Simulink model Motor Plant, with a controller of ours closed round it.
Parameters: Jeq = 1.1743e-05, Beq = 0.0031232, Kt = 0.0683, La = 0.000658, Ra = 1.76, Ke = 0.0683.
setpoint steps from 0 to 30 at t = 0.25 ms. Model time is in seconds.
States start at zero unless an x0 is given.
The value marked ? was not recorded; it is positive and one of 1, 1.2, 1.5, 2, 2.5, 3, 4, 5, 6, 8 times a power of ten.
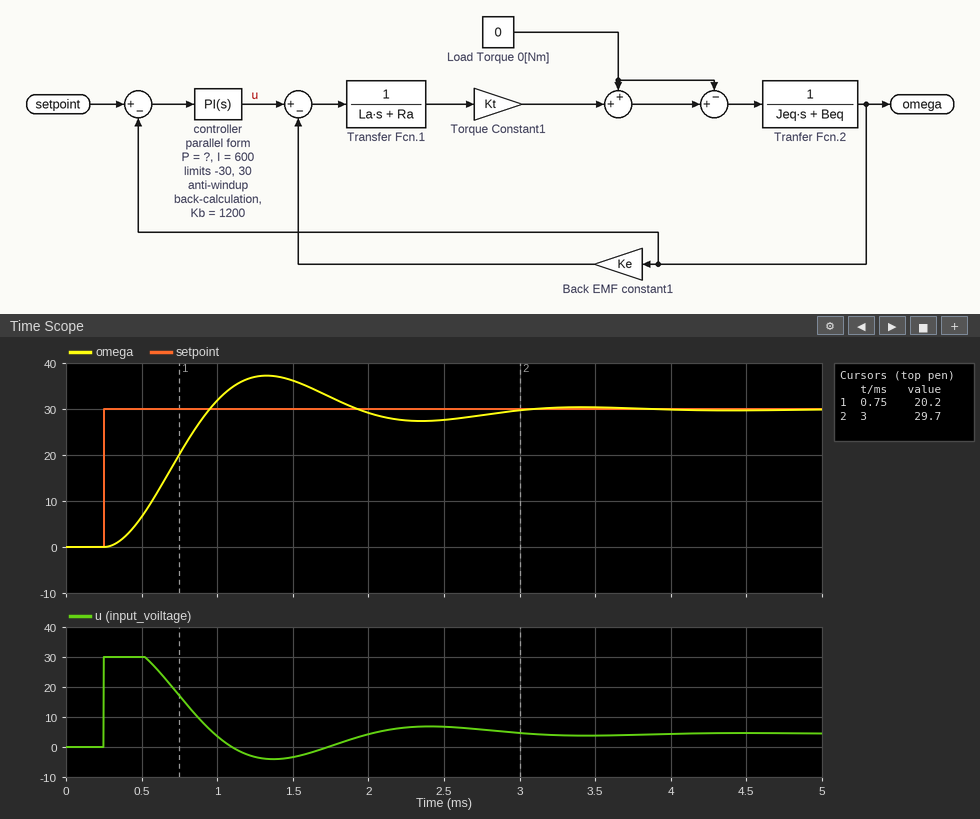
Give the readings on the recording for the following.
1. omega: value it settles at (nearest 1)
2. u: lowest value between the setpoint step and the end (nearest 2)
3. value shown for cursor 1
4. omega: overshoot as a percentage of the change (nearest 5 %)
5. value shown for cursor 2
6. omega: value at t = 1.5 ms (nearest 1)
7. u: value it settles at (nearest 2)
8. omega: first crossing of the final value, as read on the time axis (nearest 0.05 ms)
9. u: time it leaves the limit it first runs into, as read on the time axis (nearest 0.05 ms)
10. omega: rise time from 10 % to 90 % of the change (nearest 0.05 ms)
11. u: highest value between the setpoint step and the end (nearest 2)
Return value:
30
-4
20.2
25 %
29.7
36
4
0.95 ms
0.55 ms
0.45 ms
30
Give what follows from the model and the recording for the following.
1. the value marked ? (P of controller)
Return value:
1.2
